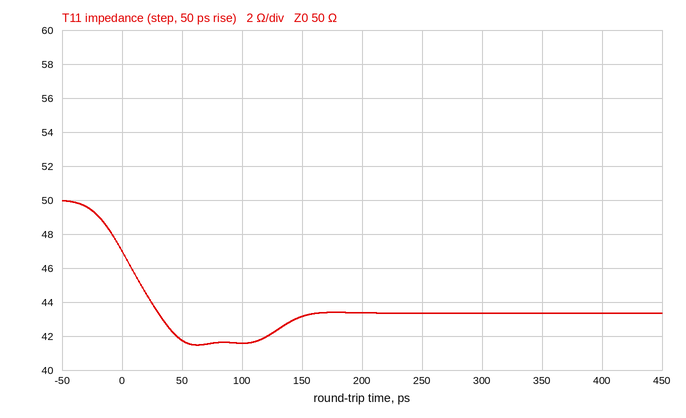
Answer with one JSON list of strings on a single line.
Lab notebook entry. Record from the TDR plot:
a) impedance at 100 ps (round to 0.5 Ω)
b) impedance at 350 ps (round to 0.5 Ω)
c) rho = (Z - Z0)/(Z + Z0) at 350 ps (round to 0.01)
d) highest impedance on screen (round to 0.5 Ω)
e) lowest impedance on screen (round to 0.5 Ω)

["41.5 Ω", "43.5 Ω", "-0.07", "50.0 Ω", "41.5 Ω"]
